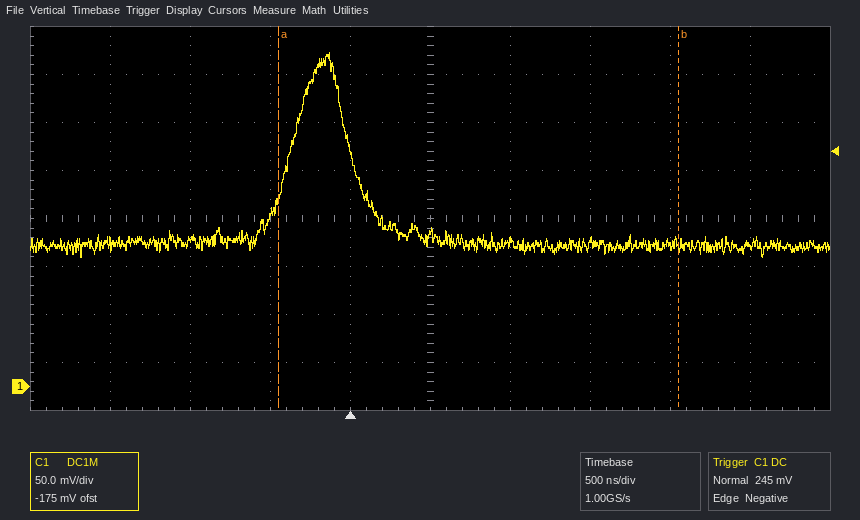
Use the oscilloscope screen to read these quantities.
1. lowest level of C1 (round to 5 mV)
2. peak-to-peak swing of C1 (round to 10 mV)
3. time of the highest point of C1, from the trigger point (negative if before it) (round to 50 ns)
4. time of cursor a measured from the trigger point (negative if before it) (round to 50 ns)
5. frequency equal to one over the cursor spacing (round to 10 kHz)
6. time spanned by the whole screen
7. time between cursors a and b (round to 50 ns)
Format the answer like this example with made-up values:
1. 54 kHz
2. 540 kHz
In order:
1. 135 mV
2. 210 mV
3. -150 ns
4. -450 ns
5. 400 kHz
6. 5 µs
7. 2.50 µs
